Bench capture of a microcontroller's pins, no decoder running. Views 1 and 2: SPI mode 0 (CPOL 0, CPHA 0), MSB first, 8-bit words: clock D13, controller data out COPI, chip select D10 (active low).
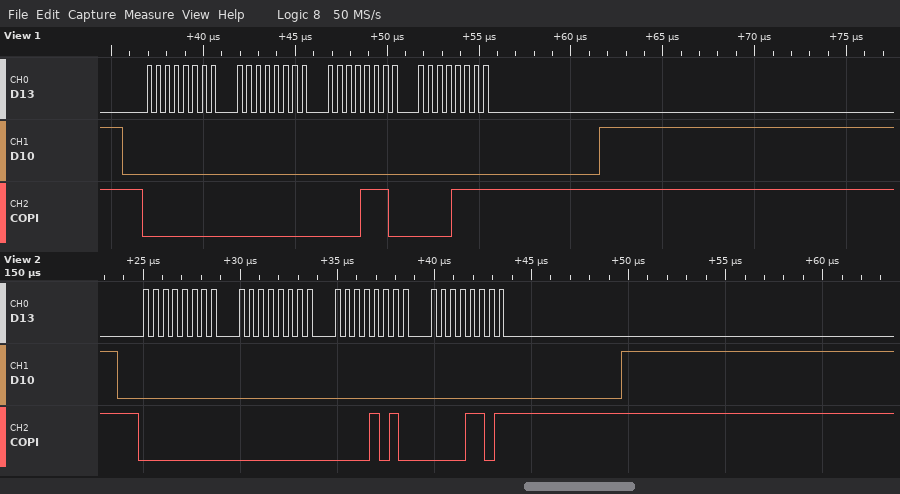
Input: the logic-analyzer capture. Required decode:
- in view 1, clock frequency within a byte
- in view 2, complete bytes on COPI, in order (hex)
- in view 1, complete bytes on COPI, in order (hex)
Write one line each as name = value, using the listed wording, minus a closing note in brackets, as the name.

in view 1, clock frequency within a byte = 2 MHz
in view 2, complete bytes on COPI, in order = 00 00 0A 0D
in view 1, complete bytes on COPI, in order = 00 00 0E 0F
